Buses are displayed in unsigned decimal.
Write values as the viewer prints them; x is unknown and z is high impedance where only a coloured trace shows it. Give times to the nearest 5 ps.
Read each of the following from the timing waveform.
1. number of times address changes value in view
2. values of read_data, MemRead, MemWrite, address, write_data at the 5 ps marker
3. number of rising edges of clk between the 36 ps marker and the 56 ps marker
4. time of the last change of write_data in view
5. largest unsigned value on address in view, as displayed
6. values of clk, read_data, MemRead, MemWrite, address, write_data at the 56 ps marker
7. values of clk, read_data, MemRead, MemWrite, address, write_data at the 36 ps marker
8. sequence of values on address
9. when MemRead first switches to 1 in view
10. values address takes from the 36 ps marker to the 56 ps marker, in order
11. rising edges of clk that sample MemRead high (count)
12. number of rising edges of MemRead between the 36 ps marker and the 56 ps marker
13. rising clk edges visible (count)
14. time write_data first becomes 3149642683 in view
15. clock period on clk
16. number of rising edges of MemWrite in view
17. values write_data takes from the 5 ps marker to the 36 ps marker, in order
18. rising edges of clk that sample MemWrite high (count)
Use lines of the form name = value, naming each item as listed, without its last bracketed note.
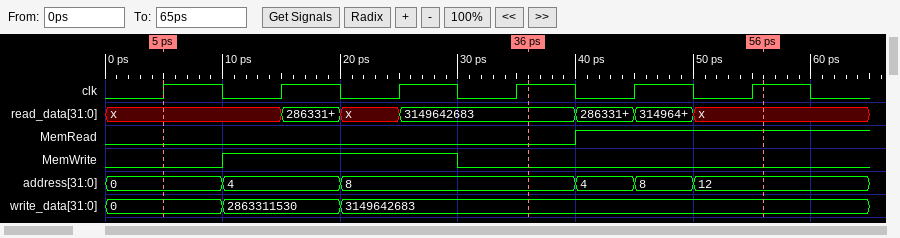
number of times address changes value in view = 5
values of read_data, MemRead, MemWrite, address, write_data at the 5 ps marker = read_data=x, MemRead=0, MemWrite=0, address=0, write_data=0
number of rising edges of clk between the 36 ps marker and the 56 ps marker = 2
time of the last change of write_data in view = 20 ps
largest unsigned value on address in view, as displayed = 12
values of clk, read_data, MemRead, MemWrite, address, write_data at the 56 ps marker = clk=1, read_data=x, MemRead=1, MemWrite=0, address=12, write_data=3149642683
values of clk, read_data, MemRead, MemWrite, address, write_data at the 36 ps marker = clk=1, read_data=3149642683, MemRead=0, MemWrite=0, address=8, write_data=3149642683
sequence of values on address = 0, 4, 8, 4, 8, 12
when MemRead first switches to 1 in view = 40 ps
values address takes from the 36 ps marker to the 56 ps marker, in order = 8, 4, 8, 12
rising edges of clk that sample MemRead high = 2
number of rising edges of MemRead between the 36 ps marker and the 56 ps marker = 1
rising clk edges visible = 6
time write_data first becomes 3149642683 in view = 20 ps
clock period on clk = 10 ps
number of rising edges of MemWrite in view = 1
values write_data takes from the 5 ps marker to the 36 ps marker, in order = 0, 2863311530, 3149642683
rising edges of clk that sample MemWrite high = 2
